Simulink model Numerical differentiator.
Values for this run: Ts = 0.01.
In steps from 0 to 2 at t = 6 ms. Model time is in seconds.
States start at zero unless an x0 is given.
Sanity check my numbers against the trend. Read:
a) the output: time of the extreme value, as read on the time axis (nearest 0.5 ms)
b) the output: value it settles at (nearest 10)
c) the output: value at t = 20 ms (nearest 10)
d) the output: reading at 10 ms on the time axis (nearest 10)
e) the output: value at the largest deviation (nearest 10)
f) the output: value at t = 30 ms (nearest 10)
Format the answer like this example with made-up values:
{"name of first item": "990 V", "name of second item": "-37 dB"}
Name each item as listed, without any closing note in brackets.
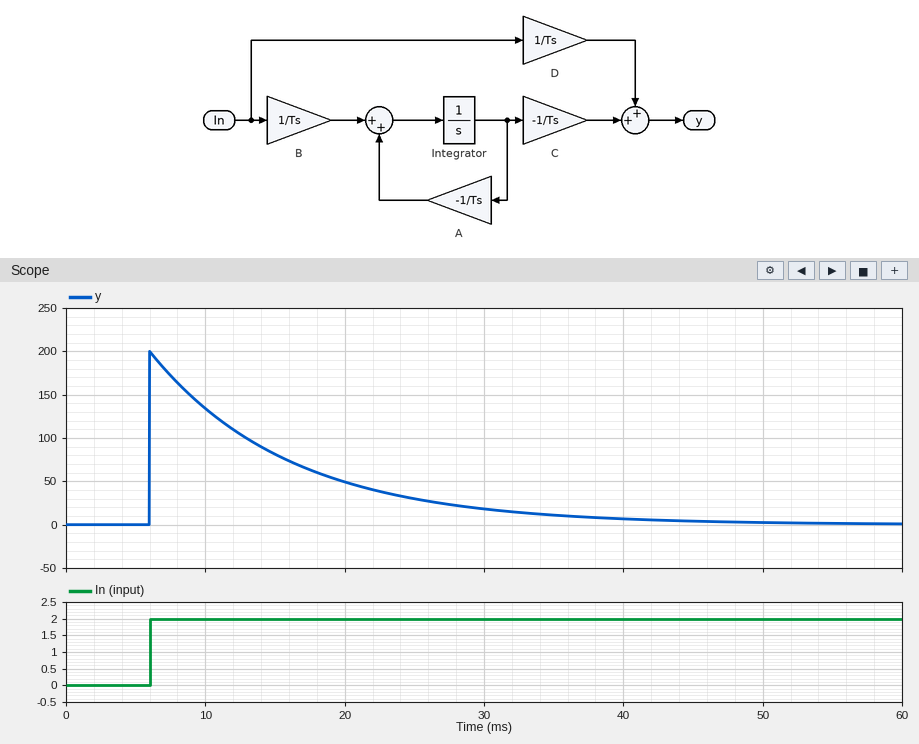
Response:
{"the output: time of the extreme value, as read on the time axis": "6.0 ms", "the output: value it settles at": "0", "the output: value at t = 20 ms": "50", "the output: reading at 10 ms on the time axis": "130", "the output: value at the largest deviation": "200", "the output: value at t = 30 ms": "20"}
